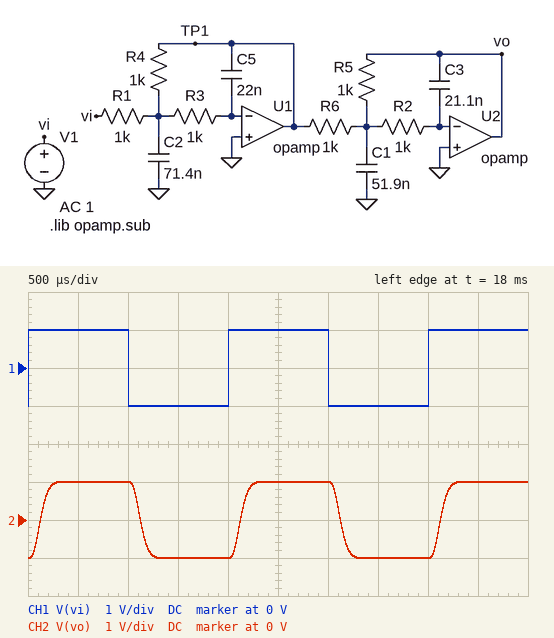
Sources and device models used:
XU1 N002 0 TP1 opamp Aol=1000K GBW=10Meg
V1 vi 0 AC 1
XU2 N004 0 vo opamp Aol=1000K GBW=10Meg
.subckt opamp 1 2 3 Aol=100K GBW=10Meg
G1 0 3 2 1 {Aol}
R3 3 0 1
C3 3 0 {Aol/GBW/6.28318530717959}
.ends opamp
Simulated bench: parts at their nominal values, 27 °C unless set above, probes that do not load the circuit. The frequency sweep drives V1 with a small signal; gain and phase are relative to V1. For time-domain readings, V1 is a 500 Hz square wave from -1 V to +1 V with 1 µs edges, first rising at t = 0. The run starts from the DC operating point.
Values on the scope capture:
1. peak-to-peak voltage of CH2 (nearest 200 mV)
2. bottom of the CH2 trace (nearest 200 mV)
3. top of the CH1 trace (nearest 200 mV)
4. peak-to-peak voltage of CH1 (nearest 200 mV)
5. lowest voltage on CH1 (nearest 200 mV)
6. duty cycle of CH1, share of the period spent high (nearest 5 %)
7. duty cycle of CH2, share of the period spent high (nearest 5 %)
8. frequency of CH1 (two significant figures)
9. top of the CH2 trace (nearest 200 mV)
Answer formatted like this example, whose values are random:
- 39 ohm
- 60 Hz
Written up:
- 2.0 V
- -1.0 V
- 1.0 V
- 2.0 V
- -1.0 V
- 50 %
- 50 %
- 500 Hz
- 1.0 V
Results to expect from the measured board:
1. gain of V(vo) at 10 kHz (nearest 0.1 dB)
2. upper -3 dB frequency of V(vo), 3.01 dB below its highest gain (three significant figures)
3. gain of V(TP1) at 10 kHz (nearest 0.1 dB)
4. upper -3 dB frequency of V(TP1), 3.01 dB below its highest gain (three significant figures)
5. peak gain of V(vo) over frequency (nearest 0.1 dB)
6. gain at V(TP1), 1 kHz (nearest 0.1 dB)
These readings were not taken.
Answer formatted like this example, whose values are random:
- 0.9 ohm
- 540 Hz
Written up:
- -30.8 dB
- 2.34 kHz
- -16.5 dB
- 3.32 kHz
- 0 dB
- -0.2 dB
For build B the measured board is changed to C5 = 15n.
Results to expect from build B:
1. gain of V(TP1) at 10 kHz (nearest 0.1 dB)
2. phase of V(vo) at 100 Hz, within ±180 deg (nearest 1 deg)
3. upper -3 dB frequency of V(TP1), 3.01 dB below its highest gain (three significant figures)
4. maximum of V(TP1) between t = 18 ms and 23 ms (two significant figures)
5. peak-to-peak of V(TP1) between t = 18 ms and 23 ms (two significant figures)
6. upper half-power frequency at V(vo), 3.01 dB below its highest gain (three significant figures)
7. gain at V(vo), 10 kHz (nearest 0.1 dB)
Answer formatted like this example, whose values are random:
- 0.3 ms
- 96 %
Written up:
- -12.7 dB
- -4 deg
- 4.99 kHz
- 1.1 V
- 2.2 V
- 3.02 kHz
- -27.0 dB
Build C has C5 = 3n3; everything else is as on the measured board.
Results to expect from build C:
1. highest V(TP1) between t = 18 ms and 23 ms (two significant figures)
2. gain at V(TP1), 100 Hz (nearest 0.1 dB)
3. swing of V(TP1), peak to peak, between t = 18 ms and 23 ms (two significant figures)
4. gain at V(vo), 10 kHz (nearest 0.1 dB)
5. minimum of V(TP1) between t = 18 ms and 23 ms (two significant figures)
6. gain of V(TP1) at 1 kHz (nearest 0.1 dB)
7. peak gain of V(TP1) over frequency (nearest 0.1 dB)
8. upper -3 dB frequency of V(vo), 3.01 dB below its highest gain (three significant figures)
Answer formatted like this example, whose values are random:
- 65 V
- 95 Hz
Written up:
- 1.7 V
- 0 dB
- 3.4 V
- -10.2 dB
- -1.7 V
- 0.1 dB
- 4.3 dB
- 3.89 kHz
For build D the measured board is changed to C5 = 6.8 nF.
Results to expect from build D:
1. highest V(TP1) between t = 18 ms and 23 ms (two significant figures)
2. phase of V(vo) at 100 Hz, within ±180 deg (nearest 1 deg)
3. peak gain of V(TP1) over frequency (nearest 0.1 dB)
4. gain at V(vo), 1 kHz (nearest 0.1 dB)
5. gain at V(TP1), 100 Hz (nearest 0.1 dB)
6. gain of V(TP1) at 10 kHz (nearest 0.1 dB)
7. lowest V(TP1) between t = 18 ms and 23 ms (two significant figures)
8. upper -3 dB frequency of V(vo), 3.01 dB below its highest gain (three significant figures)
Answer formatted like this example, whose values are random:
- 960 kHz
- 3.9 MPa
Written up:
- 1.4 V
- -3 deg
- 1.7 dB
- -0.2 dB
- 0 dB
- -4.0 dB
- -1.4 V
- 4.08 kHz
